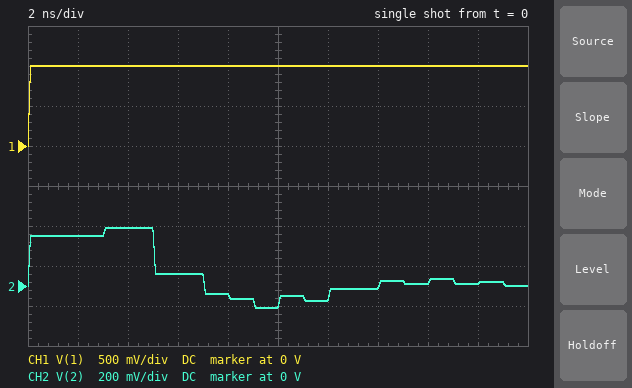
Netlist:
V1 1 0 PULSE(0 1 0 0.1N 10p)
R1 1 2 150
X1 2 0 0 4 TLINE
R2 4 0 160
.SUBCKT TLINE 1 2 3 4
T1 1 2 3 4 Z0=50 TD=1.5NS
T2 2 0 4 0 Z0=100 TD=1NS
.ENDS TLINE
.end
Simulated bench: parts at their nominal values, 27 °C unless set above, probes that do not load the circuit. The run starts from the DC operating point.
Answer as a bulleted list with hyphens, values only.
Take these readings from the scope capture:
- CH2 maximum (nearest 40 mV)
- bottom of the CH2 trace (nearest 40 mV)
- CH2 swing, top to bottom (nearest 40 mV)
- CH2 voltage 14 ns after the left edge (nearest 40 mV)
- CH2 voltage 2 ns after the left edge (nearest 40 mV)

- 280 mV
- -120 mV
- 400 mV
- 0 V
- 240 mV
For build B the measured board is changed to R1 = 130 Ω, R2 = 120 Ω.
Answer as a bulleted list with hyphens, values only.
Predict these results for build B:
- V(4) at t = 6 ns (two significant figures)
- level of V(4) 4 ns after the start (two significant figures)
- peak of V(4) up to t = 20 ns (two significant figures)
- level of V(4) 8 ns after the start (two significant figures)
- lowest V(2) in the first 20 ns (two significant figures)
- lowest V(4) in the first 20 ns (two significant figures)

- -72 mV
- -140 mV
- 53 mV
- 36 mV
- -86 mV
- -290 mV
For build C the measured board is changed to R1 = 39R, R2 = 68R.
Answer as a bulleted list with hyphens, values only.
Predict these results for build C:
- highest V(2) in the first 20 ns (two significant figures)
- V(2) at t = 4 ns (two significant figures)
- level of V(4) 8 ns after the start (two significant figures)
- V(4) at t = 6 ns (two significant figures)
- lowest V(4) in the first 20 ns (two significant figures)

- 560 mV
- 510 mV
- -110 mV
- -160 mV
- -500 mV
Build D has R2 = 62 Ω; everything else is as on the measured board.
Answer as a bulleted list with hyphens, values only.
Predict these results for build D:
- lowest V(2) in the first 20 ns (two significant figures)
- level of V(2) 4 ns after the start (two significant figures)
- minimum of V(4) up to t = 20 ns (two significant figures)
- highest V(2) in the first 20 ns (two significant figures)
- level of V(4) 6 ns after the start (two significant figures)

- -44 mV
- 200 mV
- -220 mV
- 250 mV
- -55 mV
